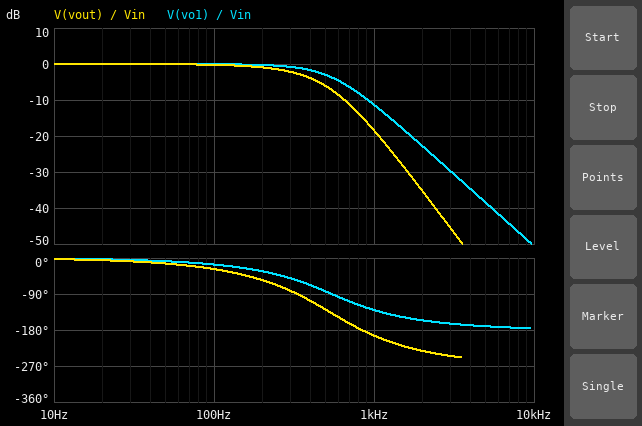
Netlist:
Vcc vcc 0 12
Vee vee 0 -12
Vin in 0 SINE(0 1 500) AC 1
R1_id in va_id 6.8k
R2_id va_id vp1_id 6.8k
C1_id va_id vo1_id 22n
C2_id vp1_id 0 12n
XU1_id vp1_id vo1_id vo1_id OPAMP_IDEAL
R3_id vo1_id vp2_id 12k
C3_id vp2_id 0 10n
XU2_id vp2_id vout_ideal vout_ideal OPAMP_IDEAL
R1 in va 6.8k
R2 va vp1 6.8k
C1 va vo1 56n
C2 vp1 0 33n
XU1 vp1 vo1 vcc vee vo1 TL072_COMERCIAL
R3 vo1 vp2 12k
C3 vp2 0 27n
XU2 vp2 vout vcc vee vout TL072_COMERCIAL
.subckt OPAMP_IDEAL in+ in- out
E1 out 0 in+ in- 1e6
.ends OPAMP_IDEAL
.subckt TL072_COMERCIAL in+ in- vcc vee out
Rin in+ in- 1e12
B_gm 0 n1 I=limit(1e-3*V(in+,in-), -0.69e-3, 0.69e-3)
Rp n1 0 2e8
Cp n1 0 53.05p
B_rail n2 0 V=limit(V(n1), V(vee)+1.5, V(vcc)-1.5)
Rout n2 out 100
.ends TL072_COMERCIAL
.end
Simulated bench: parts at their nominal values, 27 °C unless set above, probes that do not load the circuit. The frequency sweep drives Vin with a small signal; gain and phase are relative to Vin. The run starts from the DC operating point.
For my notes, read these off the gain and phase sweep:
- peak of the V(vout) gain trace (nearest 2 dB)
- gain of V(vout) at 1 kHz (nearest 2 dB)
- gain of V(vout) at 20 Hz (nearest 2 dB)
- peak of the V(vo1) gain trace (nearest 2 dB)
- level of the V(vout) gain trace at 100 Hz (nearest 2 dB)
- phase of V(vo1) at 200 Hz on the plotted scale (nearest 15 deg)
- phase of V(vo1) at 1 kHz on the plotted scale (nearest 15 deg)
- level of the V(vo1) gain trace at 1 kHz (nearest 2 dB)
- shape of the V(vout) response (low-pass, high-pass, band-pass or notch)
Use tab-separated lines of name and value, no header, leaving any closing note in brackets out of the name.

peak of the V(vout) gain trace	0 dB
gain of V(vout) at 1 kHz	-18 dB
gain of V(vout) at 20 Hz	0 dB
peak of the V(vo1) gain trace	0 dB
level of the V(vout) gain trace at 100 Hz	0 dB
phase of V(vo1) at 200 Hz on the plotted scale	-30 deg
phase of V(vo1) at 1 kHz on the plotted scale	-135 deg
level of the V(vo1) gain trace at 1 kHz	-12 dB
shape of the V(vout) response	low-pass
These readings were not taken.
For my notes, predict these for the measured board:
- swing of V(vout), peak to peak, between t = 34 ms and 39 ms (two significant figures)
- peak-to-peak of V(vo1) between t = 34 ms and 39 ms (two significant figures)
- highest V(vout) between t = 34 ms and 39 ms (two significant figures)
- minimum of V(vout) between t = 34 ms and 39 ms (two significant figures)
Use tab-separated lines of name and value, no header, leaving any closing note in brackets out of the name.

swing of V(vout), peak to peak, between t = 34 ms and 39 ms	990 mV
peak-to-peak of V(vo1) between t = 34 ms and 39 ms	1.4 V
highest V(vout) between t = 34 ms and 39 ms	490 mV
minimum of V(vout) between t = 34 ms and 39 ms	-490 mV
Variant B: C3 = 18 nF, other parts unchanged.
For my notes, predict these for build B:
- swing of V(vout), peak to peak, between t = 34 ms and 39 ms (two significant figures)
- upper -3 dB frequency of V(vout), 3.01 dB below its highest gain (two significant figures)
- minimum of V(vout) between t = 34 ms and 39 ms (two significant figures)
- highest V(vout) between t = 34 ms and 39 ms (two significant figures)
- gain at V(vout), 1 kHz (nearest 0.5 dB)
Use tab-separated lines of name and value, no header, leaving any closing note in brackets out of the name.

swing of V(vout), peak to peak, between t = 34 ms and 39 ms	1.2 V
upper -3 dB frequency of V(vout), 3.01 dB below its highest gain	410 Hz
minimum of V(vout) between t = 34 ms and 39 ms	-580 mV
highest V(vout) between t = 34 ms and 39 ms	580 mV
gain at V(vout), 1 kHz	-16.0 dB
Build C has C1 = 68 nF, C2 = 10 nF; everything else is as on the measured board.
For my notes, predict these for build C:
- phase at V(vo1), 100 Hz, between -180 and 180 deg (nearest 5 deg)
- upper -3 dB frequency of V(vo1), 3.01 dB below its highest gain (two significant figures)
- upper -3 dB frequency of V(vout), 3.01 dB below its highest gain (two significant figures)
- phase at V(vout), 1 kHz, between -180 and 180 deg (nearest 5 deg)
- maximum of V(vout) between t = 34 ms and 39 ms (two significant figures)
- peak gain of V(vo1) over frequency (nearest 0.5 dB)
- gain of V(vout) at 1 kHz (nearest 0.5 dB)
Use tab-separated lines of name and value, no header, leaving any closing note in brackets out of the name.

phase at V(vo1), 100 Hz, between -180 and 180 deg	-5 deg
upper -3 dB frequency of V(vo1), 3.01 dB below its highest gain	1.1 kHz
upper -3 dB frequency of V(vout), 3.01 dB below its highest gain	830 Hz
phase at V(vout), 1 kHz, between -180 and 180 deg	-170 deg
maximum of V(vout) between t = 34 ms and 39 ms	860 mV
peak gain of V(vo1) over frequency	3.0 dB
gain of V(vout) at 1 kHz	-6.0 dB
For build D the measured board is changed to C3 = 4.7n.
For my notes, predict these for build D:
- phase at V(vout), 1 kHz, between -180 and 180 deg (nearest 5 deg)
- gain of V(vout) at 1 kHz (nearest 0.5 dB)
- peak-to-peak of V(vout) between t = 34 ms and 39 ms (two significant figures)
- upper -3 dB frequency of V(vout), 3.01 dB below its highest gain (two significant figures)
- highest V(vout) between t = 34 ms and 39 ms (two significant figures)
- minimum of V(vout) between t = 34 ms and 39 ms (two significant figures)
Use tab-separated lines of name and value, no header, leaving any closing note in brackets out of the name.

phase at V(vout), 1 kHz, between -180 and 180 deg	-150 deg
gain of V(vout) at 1 kHz	-12.0 dB
peak-to-peak of V(vout) between t = 34 ms and 39 ms	1.4 V
upper -3 dB frequency of V(vout), 3.01 dB below its highest gain	490 Hz
highest V(vout) between t = 34 ms and 39 ms	690 mV
minimum of V(vout) between t = 34 ms and 39 ms	-690 mV
